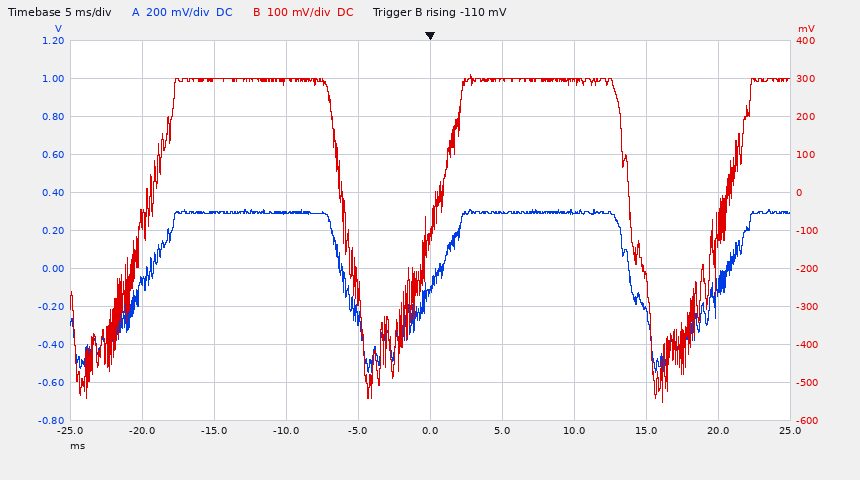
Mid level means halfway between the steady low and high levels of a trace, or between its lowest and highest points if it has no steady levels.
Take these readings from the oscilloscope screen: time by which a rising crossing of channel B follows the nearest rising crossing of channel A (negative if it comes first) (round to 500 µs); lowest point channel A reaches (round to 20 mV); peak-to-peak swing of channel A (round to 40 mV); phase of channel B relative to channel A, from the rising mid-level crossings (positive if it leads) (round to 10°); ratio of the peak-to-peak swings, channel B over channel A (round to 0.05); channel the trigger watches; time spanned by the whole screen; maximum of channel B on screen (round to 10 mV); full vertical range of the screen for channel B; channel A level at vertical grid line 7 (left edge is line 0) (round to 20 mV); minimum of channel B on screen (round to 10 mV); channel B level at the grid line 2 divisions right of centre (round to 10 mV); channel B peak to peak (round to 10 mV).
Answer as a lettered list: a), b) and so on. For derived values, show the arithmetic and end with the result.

a) 0.0 ms
b) -540 mV
c) 840 mV
d) 0°
e) 860 mV / 840 mV ≈ 1.02, so 1.00 to the nearest 0.05
f) channel B
g) 50 ms
h) 310 mV
i) 1 V
j) 300 mV
k) -550 mV
l) 290 mV
m) 310 mV − (-550 mV) = 860 mV
